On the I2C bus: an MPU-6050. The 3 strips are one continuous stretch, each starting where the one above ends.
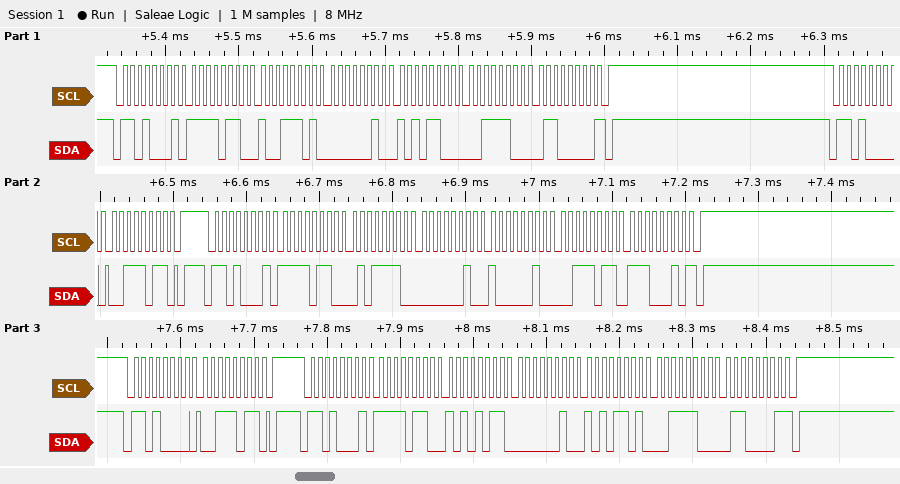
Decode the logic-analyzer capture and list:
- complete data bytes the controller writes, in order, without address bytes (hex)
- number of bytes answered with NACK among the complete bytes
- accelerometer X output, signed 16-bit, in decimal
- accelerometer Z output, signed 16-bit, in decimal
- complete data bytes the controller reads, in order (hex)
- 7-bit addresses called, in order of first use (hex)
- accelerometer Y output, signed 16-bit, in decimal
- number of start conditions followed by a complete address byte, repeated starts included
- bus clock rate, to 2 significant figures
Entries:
3B 3B
3
-2466
15330
F6 9D 02 AC 3C 60 F6 5E 02 82 3B E2 F6 AB 02 AD 3C 61
0x68
642
5
100 kHz
